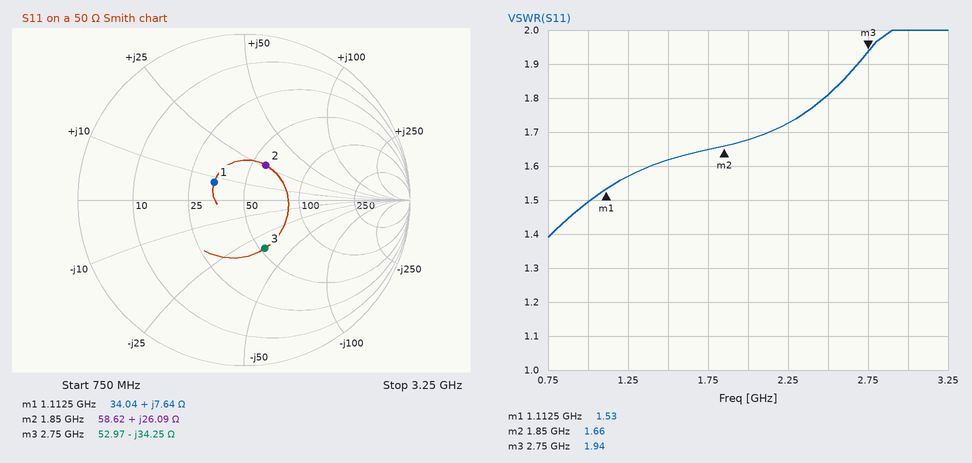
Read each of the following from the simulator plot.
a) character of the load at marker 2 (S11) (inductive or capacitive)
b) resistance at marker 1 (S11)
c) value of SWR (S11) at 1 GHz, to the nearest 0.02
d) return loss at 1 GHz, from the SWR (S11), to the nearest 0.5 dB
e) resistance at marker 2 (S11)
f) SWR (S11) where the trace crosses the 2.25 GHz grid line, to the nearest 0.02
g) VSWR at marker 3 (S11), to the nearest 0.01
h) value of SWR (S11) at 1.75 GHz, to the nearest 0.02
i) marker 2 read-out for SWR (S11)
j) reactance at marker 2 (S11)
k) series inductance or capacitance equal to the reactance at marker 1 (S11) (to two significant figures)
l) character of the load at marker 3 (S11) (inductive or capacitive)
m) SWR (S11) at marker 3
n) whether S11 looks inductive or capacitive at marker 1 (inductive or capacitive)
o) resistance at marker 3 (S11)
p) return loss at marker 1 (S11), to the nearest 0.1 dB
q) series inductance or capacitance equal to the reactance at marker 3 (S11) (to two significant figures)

inductive
34.04 Ω
1.50
14.0 dB
58.62 Ω
1.72
1.93
1.64
1.66
+26.09 Ω
1.1 nH
capacitive
1.94
inductive
52.97 Ω
13.6 dB
1.7 pF
